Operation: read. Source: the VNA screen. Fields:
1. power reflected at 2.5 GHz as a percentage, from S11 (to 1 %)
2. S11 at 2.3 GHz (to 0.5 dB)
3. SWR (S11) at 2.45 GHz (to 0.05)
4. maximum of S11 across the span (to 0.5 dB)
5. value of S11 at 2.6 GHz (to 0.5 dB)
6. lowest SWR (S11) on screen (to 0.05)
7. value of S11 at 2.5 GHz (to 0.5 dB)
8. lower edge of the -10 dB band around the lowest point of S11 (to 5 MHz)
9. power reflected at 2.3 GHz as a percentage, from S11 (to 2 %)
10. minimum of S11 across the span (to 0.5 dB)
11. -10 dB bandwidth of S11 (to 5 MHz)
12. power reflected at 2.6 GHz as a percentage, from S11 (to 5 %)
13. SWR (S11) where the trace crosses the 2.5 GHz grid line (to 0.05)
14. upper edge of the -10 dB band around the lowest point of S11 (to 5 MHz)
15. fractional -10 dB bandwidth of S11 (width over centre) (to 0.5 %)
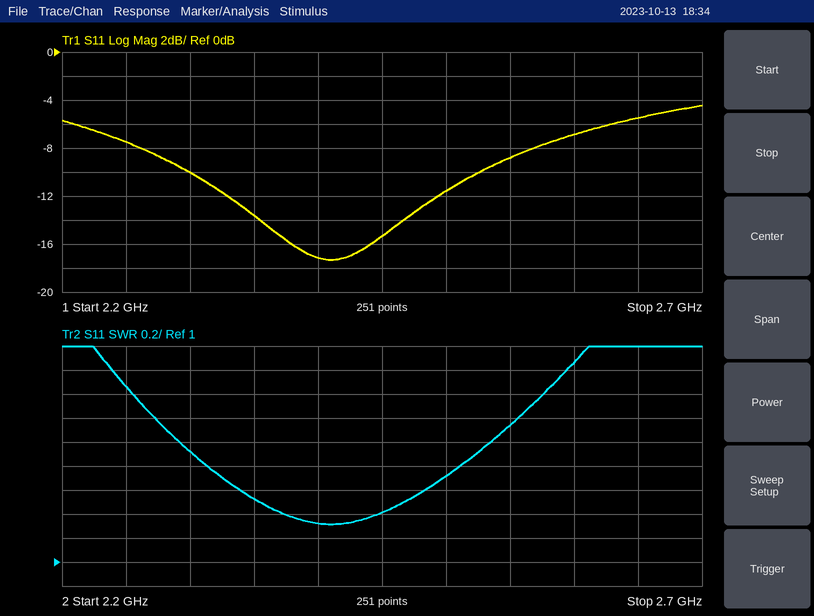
7 %
-10.0 dB
1.40
-4.5 dB
-7.0 dB
1.30
-11.5 dB
2.300 GHz
10 %
-17.5 dB
225 MHz
20 %
1.70
2.525 GHz
9.5 %
